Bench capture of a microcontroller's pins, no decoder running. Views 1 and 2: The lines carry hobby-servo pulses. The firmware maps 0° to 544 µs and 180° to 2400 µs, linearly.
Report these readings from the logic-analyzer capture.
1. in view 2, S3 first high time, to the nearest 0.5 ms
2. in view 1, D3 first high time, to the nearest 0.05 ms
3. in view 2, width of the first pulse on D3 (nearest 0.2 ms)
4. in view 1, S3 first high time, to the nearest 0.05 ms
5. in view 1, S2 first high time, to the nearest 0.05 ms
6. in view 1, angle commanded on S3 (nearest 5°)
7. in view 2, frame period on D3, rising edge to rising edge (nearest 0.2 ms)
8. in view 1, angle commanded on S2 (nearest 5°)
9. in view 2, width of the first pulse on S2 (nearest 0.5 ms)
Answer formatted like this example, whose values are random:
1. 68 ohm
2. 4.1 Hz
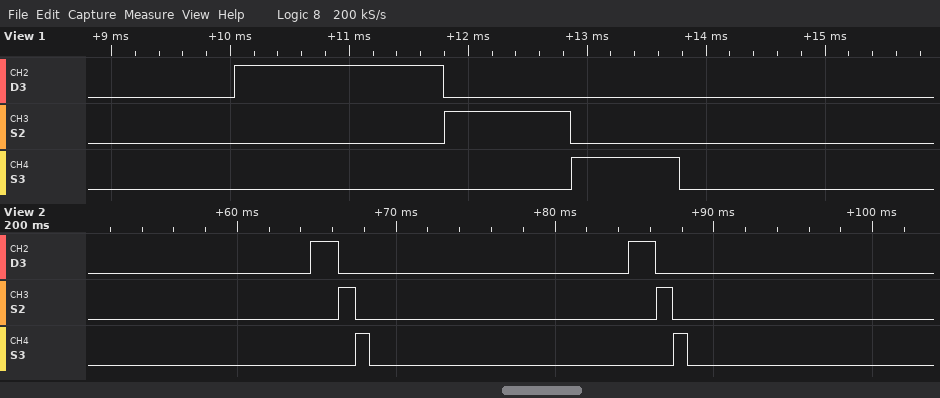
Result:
1. 1.0 ms
2. 1.75 ms
3. 1.8 ms
4. 0.90 ms
5. 1.05 ms
6. 35°
7. 20.0 ms
8. 50°
9. 1.0 ms
